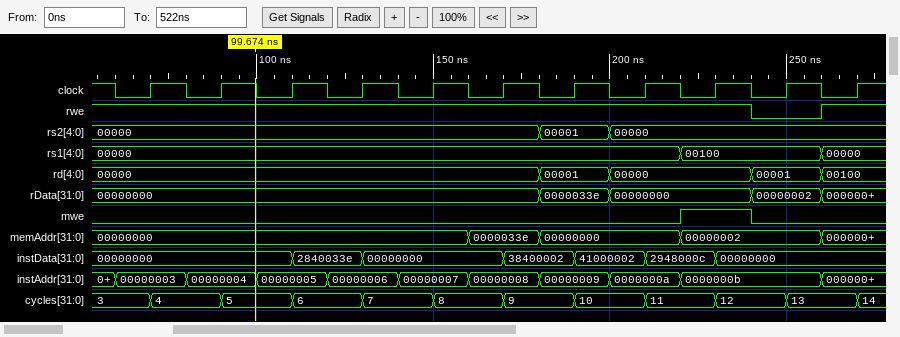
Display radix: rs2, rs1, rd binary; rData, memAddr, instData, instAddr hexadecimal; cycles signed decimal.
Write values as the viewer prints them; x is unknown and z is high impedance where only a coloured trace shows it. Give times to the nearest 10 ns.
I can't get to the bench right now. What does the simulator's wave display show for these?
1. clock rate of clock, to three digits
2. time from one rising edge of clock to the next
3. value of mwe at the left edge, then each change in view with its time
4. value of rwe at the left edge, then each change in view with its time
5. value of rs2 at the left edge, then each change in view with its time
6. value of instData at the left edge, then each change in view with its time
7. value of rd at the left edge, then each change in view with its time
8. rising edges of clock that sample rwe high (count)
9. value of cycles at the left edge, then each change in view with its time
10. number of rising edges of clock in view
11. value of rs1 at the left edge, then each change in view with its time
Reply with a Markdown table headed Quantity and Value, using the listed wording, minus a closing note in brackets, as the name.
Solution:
| Quantity | Value |
|---|---|
| clock rate of clock, to three digits | 50.0 MHz |
| time from one rising edge of clock to the next | 20 ns |
| value of mwe at the left edge, then each change in view with its time | 0, 1 at 220 ns, 0 at 240 ns |
| value of rwe at the left edge, then each change in view with its time | 1, 0 at 240 ns, 1 at 260 ns |
| value of rs2 at the left edge, then each change in view with its time | 00000, 00001 at 180 ns, 00000 at 200 ns |
| value of instData at the left edge, then each change in view with its time | 00000000, 2840033e at 110 ns, 00000000 at 130 ns, 38400002 at 170 ns, 41000002 at 190 ns, 2948000c at 210 ns, 00000000 at 230 ns |
| value of rd at the left edge, then each change in view with its time | 00000, 00001 at 180 ns, 00000 at 200 ns, 00001 at 240 ns, 00100 at 260 ns |
| rising edges of clock that sample rwe high | 10 |
| value of cycles at the left edge, then each change in view with its time | 3, 4 at 70 ns, 5 at 90 ns, 6 at 110 ns, 7 at 130 ns, 8 at 150 ns, 9 at 170 ns, 10 at 190 ns, 11 at 210 ns, 12 at 230 ns, 13 at 250 ns, 14 at 270 ns |
| number of rising edges of clock in view | 11 |
| value of rs1 at the left edge, then each change in view with its time | 00000, 00100 at 220 ns, 00000 at 260 ns |
